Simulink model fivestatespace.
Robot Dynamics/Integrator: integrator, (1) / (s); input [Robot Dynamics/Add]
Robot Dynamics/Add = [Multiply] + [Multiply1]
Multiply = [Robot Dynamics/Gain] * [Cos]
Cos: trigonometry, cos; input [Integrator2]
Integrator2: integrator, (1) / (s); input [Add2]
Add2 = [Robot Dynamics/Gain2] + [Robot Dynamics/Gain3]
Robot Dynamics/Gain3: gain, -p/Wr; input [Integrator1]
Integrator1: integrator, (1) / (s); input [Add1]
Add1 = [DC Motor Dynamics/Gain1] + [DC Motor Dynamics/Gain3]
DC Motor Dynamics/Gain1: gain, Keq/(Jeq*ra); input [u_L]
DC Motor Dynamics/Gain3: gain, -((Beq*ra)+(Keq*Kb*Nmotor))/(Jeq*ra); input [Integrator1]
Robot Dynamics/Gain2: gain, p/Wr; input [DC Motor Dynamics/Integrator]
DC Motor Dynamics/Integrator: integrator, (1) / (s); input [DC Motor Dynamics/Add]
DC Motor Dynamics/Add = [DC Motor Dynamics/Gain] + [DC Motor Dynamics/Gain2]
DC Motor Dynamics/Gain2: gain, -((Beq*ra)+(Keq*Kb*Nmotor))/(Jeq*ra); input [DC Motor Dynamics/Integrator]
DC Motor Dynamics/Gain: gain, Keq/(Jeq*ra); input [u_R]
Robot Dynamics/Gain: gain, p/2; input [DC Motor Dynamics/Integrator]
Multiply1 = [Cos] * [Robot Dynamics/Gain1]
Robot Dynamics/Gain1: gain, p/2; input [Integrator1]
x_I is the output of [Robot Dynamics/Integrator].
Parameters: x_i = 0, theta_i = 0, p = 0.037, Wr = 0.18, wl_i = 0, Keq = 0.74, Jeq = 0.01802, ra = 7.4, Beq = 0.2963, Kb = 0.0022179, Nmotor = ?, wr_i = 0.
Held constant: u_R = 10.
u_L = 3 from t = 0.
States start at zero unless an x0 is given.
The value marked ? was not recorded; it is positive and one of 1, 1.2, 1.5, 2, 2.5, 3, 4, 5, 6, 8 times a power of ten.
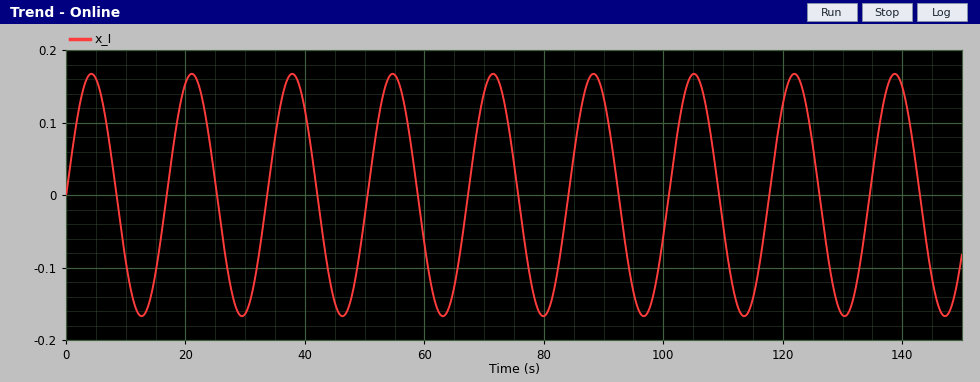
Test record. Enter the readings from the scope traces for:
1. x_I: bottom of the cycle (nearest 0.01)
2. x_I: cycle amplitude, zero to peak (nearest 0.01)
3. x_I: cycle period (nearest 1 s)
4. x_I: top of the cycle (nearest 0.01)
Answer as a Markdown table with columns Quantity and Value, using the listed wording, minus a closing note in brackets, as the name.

| Quantity | Value |
|---|---|
| x_I: bottom of the cycle | -0.17 |
| x_I: cycle amplitude, zero to peak | 0.17 |
| x_I: cycle period | 17 s |
| x_I: top of the cycle | 0.17 |
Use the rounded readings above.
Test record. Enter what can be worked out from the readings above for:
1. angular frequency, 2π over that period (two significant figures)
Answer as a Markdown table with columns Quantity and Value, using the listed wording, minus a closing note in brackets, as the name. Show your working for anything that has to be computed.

| Quantity | Value |
|---|---|
| angular frequency, 2π over that period | 2π / 17 = 0.37 rad/s |
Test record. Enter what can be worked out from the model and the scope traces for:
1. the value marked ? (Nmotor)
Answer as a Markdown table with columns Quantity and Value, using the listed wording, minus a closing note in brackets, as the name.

| Quantity | Value |
|---|---|
| the value marked ? | 400 |
